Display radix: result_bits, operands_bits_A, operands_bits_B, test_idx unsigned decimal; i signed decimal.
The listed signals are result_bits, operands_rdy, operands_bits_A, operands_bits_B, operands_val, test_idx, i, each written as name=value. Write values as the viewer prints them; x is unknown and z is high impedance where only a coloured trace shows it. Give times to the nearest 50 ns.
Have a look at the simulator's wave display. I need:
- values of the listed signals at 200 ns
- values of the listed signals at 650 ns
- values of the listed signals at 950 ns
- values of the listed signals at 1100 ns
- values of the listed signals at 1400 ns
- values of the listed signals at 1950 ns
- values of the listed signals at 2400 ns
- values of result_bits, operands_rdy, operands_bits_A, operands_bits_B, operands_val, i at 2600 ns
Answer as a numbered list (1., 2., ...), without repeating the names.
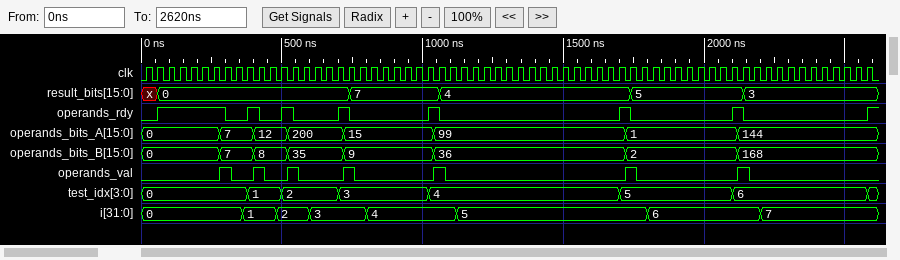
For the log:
1. result_bits=0, operands_rdy=1, operands_bits_A=0, operands_bits_B=0, operands_val=0, test_idx=0, i=0
2. result_bits=0, operands_rdy=0, operands_bits_A=200, operands_bits_B=35, operands_val=0, test_idx=2, i=3
3. result_bits=7, operands_rdy=0, operands_bits_A=15, operands_bits_B=9, operands_val=0, test_idx=3, i=4
4. result_bits=4, operands_rdy=0, operands_bits_A=99, operands_bits_B=36, operands_val=0, test_idx=4, i=4
5. result_bits=4, operands_rdy=0, operands_bits_A=99, operands_bits_B=36, operands_val=0, test_idx=4, i=5
6. result_bits=5, operands_rdy=0, operands_bits_A=1, operands_bits_B=2, operands_val=0, test_idx=5, i=6
7. result_bits=3, operands_rdy=0, operands_bits_A=144, operands_bits_B=168, operands_val=0, test_idx=6, i=7
8. result_bits=3, operands_rdy=1, operands_bits_A=144, operands_bits_B=168, operands_val=0, i=7
